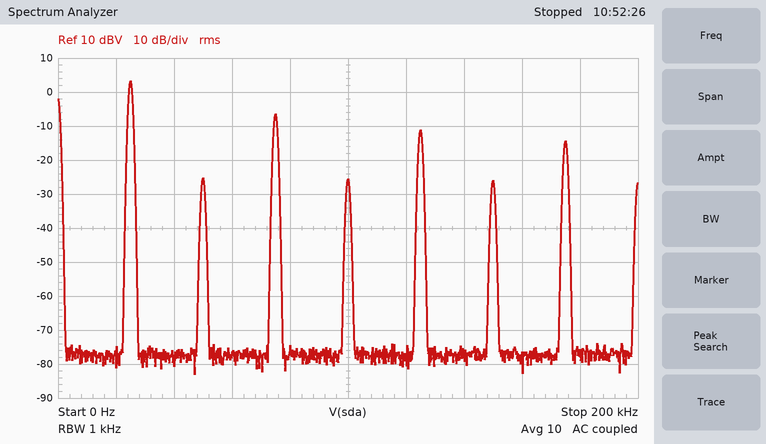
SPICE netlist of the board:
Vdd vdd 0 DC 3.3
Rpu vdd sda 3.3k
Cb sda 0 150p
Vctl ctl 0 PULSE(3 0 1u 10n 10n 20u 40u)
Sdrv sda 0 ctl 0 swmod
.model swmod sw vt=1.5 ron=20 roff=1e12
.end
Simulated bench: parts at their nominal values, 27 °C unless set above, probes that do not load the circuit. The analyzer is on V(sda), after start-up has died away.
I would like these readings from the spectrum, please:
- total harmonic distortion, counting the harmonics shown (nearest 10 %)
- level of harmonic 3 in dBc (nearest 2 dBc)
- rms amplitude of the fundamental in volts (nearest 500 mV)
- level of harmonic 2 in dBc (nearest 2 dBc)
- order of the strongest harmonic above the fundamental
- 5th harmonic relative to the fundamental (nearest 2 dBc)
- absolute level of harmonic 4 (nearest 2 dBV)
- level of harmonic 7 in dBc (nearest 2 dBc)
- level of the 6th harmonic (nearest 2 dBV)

40 %
-10 dBc
1.5 V
-28 dBc
3
-14 dBc
-26 dBV
-18 dBc
-26 dBV
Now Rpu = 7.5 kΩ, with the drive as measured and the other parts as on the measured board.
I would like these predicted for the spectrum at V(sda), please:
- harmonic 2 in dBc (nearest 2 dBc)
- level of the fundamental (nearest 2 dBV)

-22 dBc
4 dBV
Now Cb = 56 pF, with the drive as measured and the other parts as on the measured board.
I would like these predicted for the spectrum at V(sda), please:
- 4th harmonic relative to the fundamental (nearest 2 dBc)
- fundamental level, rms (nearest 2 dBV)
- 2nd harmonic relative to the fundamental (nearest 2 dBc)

-38 dBc
4 dBV
-38 dBc
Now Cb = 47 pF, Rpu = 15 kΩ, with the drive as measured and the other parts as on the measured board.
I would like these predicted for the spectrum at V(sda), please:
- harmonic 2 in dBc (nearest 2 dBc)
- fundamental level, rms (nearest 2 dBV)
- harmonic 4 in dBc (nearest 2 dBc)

-26 dBc
4 dBV
-26 dBc
